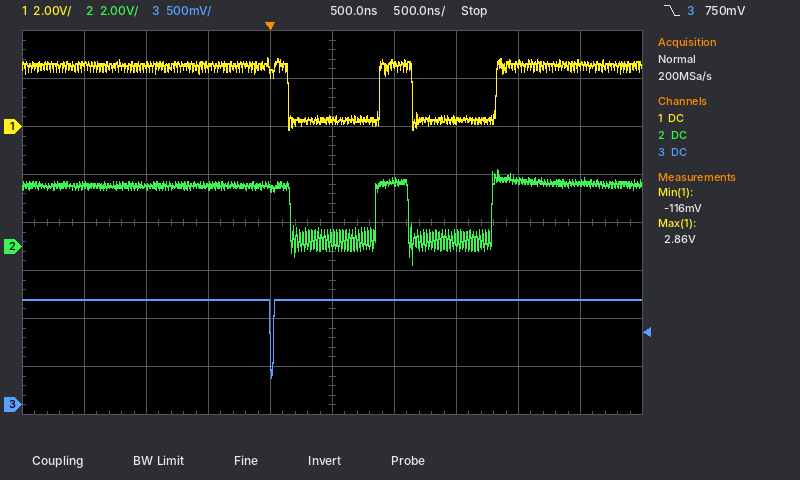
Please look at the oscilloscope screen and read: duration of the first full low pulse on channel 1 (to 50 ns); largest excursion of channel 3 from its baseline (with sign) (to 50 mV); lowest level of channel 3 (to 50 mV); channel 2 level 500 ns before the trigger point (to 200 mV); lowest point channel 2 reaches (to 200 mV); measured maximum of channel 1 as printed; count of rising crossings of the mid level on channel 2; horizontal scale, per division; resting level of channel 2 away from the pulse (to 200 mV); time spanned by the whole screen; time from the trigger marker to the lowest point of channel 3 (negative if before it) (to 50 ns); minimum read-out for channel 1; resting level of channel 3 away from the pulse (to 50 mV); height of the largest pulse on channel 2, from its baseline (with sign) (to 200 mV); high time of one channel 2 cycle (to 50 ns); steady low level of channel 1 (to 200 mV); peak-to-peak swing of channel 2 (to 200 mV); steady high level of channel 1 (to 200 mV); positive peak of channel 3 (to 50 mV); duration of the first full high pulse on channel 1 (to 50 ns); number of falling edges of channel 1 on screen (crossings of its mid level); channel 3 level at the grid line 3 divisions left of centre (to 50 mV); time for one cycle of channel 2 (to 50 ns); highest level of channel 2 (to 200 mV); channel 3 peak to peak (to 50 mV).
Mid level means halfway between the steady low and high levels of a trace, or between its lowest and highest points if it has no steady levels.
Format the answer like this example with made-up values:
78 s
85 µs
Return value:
750 ns
-800 mV
300 mV
2.6 V
-800 mV
2.86 V
2
500 ns
2.6 V
5 µs
0 ns
-116 mV
1.10 V
-3.4 V
250 ns
200 mV
4.0 V
2.6 V
1.10 V
250 ns
2
1.10 V
950 ns
3.2 V
800 mV
